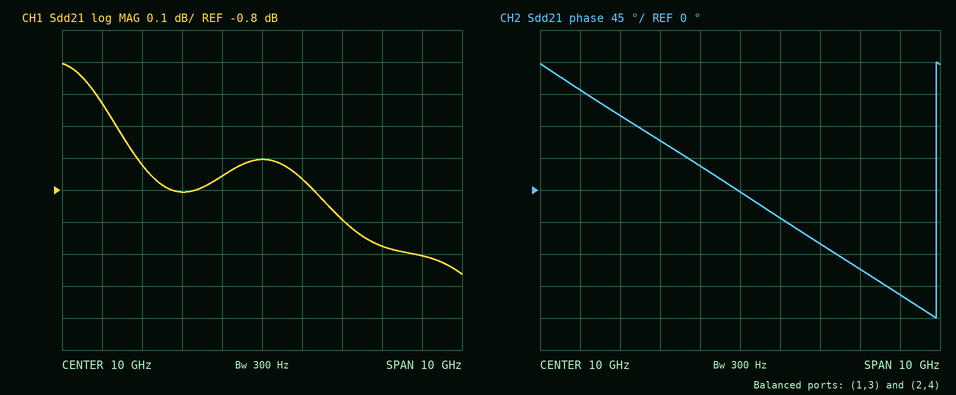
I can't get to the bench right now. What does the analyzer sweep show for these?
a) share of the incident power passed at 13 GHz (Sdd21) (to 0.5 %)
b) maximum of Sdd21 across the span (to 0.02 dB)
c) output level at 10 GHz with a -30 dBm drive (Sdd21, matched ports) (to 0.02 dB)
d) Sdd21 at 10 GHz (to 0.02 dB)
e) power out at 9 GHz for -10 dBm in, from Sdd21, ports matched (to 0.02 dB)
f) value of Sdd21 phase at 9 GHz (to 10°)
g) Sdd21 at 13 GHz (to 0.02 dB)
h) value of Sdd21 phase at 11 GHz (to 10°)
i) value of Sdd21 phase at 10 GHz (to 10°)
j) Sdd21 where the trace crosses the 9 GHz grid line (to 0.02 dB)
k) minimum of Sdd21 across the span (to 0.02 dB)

80.0 %
-0.40 dB
-30.70 dBm
-0.70 dB
-10.76 dBm
30°
-0.98 dB
-40°
0°
-0.76 dB
-1.06 dB
